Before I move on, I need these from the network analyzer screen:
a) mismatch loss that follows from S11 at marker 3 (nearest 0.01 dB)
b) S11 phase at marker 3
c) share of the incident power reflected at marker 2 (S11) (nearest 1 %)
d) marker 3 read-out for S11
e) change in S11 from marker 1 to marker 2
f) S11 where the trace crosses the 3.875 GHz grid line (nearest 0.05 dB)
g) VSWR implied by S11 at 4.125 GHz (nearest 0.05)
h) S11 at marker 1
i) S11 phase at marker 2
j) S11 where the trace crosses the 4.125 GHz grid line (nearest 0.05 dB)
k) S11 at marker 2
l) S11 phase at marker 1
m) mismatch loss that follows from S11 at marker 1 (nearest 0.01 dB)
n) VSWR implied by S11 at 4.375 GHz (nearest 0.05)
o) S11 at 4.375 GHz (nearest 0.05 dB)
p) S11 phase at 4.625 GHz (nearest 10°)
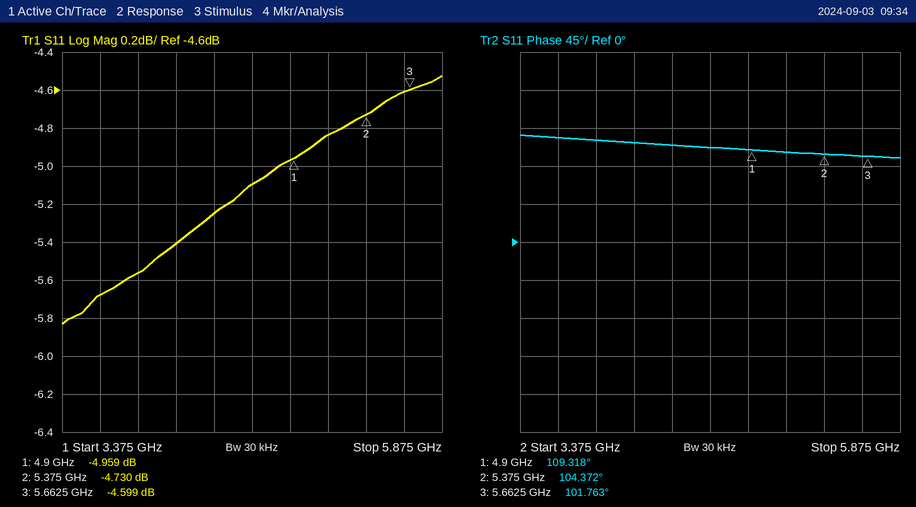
1.85 dB
101.763°
34 %
-4.599 dB
0.229 dB
-5.55 dB
3.30
-4.959 dB
104.372°
-5.40 dB
-4.730 dB
109.318°
1.67 dB
3.40
-5.25 dB
110°
